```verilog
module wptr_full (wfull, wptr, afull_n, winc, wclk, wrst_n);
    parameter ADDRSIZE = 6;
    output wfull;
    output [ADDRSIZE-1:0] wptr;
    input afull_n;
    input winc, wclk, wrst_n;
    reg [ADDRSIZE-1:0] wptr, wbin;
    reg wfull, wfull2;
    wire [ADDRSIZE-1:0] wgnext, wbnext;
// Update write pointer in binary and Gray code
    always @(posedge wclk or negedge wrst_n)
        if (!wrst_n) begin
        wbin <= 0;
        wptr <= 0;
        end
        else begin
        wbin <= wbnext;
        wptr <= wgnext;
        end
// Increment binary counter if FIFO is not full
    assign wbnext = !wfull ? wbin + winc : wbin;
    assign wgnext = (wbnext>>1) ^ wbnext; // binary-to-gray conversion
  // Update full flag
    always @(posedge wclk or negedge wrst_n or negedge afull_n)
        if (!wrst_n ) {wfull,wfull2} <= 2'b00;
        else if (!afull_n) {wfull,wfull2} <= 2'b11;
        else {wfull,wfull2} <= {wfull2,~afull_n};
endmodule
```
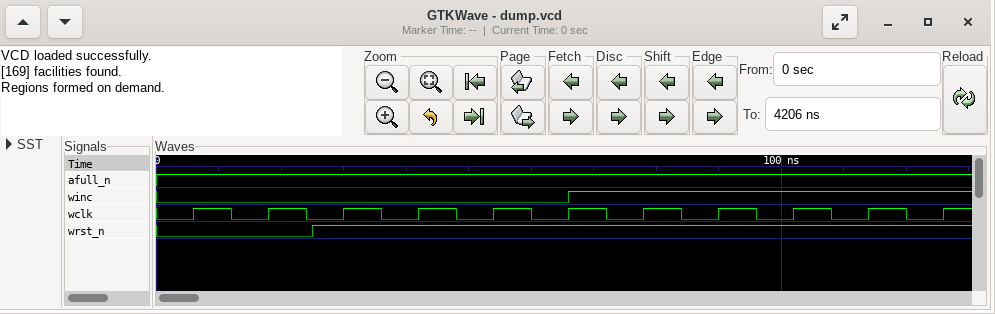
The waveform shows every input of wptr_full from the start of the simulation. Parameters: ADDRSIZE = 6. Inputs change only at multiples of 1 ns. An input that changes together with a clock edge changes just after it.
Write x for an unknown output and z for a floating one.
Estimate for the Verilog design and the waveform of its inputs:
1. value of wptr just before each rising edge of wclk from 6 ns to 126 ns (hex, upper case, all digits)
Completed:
00, 00, 00, 00, 00, 00, 00, 01, 03, 02, 06
